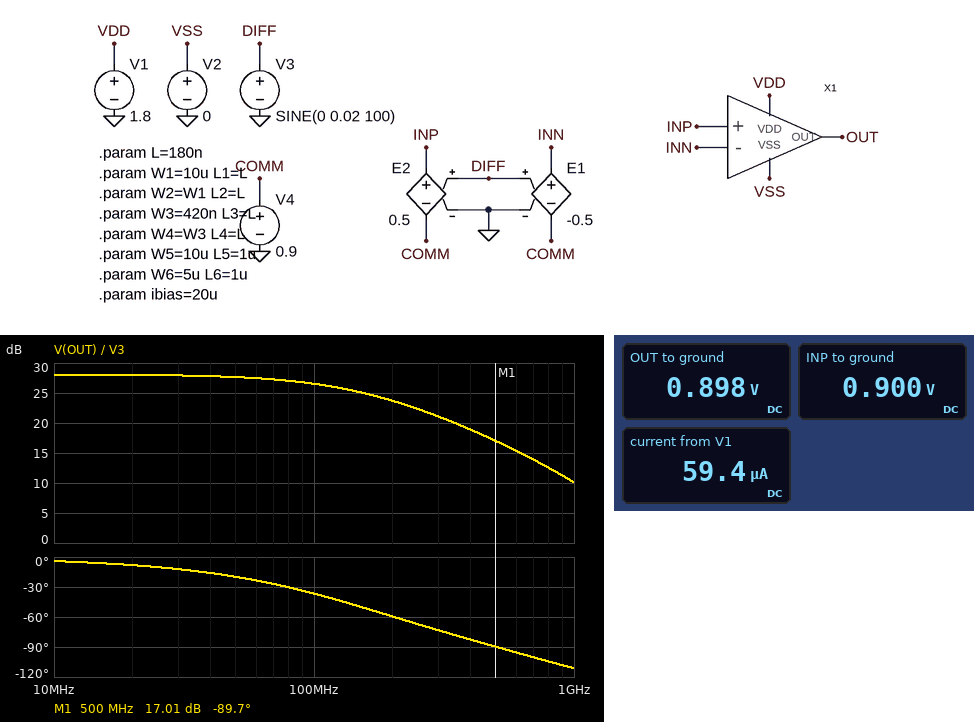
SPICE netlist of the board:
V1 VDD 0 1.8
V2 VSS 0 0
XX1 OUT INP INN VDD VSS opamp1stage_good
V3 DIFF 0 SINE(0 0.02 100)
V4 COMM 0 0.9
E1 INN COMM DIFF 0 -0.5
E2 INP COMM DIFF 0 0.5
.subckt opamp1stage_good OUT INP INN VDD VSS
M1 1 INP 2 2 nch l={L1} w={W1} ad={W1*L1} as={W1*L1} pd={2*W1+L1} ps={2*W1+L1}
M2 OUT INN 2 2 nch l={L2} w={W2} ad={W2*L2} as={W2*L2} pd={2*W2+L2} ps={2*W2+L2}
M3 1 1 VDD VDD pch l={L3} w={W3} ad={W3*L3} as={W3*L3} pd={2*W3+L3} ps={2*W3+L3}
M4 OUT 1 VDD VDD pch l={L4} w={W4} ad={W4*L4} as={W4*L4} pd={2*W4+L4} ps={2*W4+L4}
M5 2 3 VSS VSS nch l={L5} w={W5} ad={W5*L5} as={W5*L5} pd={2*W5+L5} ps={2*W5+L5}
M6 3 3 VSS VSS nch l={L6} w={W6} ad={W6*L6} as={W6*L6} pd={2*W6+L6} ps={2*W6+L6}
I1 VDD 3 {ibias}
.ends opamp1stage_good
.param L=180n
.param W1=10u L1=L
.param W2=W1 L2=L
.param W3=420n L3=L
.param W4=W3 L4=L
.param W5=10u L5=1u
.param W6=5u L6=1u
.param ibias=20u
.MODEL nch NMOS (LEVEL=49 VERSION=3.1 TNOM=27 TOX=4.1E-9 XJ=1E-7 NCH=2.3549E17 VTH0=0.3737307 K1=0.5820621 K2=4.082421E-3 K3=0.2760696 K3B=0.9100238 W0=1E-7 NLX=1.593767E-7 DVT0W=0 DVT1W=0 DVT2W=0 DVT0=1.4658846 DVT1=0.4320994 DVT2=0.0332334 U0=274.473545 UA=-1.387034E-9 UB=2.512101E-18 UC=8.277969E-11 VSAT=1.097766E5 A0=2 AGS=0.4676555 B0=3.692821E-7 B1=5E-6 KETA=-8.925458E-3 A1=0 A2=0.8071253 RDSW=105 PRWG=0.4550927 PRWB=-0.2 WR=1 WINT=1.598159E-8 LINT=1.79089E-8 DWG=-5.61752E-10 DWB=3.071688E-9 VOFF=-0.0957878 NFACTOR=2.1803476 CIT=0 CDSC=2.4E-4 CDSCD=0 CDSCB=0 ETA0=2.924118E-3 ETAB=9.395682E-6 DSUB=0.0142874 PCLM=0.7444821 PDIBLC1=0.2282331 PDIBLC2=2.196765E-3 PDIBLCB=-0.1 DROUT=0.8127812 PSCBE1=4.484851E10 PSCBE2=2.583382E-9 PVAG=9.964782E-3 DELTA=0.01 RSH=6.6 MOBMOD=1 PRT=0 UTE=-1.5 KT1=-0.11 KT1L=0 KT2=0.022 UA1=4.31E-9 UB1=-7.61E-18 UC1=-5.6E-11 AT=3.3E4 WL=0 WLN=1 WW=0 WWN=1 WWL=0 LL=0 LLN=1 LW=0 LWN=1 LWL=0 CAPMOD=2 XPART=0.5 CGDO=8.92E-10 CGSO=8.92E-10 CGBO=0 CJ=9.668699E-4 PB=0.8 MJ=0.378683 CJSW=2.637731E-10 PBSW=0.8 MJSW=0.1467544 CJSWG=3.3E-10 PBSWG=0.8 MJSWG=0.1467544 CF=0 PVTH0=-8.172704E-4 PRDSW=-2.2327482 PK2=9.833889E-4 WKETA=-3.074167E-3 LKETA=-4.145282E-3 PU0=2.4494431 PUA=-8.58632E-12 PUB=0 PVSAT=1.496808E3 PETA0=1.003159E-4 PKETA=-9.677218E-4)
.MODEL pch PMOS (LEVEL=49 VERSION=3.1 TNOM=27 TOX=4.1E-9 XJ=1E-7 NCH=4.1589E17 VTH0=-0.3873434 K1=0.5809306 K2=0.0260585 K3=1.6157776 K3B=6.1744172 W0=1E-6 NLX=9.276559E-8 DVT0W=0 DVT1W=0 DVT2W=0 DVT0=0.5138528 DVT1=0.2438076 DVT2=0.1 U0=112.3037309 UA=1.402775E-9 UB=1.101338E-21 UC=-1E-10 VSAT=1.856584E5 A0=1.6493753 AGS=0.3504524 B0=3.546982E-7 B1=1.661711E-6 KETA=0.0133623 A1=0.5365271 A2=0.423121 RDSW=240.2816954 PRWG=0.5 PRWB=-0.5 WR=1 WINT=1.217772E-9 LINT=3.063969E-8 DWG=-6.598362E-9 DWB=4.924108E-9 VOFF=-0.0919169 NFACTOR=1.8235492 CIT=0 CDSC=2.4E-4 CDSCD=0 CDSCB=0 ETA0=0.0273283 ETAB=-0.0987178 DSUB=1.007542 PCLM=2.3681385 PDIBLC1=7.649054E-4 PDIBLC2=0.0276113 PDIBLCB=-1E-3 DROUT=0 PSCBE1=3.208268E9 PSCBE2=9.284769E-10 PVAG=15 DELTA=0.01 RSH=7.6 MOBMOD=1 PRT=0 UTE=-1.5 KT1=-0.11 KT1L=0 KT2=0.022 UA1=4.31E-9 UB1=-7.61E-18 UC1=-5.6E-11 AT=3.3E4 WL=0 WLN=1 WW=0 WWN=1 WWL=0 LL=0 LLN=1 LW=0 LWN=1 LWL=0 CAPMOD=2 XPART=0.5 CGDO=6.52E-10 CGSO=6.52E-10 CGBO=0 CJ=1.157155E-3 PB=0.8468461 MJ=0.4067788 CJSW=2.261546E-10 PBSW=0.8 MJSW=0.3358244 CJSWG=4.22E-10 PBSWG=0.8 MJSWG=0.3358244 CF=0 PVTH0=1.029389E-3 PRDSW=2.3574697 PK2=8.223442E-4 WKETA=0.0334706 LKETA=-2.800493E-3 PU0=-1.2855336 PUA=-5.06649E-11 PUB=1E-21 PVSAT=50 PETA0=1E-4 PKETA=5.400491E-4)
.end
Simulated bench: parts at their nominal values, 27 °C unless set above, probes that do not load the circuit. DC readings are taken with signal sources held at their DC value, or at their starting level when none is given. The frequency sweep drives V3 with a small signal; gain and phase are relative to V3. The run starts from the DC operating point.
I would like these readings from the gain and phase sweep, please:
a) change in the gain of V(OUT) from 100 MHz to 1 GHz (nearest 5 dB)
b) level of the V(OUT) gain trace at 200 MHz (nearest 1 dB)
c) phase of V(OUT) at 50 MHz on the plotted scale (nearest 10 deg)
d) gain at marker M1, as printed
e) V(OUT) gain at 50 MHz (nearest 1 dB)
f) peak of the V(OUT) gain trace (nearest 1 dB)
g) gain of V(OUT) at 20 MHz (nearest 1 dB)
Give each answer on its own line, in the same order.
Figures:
-15 dB
24 dB
-20 deg
17.01 dB
28 dB
28 dB
28 dB
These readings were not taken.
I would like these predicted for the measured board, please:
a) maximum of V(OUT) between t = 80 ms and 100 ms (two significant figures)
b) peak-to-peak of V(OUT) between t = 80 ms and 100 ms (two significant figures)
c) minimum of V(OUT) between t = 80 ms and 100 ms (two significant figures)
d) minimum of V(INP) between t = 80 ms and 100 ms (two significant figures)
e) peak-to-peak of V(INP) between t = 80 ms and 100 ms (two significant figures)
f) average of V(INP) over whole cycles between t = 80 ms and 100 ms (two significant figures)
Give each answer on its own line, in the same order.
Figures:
1.4 V
890 mV
490 mV
890 mV
20 mV
900 mV
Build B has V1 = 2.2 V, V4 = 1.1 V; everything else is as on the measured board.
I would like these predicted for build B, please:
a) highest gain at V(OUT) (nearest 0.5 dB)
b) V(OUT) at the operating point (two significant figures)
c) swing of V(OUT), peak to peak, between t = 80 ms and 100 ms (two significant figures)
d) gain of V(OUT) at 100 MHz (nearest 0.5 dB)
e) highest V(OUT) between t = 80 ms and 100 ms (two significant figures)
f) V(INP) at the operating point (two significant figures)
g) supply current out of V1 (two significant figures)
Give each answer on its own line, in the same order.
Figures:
28.5 dB
1.3 V
1.0 V
27.0 dB
1.8 V
1.1 V
60 µA
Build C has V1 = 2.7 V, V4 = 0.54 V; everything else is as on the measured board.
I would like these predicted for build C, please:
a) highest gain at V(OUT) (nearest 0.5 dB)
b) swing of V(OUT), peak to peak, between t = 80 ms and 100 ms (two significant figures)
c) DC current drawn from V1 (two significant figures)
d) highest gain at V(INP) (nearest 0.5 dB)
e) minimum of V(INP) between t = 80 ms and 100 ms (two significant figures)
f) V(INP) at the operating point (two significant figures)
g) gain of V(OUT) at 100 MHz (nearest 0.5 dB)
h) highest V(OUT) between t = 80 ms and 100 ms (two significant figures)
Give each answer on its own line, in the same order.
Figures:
30.0 dB
1.2 V
51 µA
-6.0 dB
530 mV
540 mV
27.0 dB
2.4 V
